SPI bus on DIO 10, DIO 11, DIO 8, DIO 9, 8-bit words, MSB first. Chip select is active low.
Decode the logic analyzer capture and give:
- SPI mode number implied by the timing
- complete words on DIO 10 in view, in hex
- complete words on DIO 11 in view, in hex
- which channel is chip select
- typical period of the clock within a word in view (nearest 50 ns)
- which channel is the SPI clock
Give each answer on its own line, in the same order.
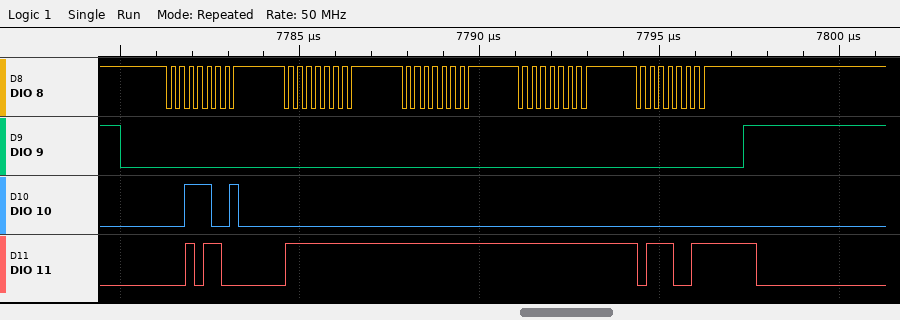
3
39, 00, 00, 00, 00
2C, FF, FF, FF, 73
DIO 9
250 ns
DIO 8
